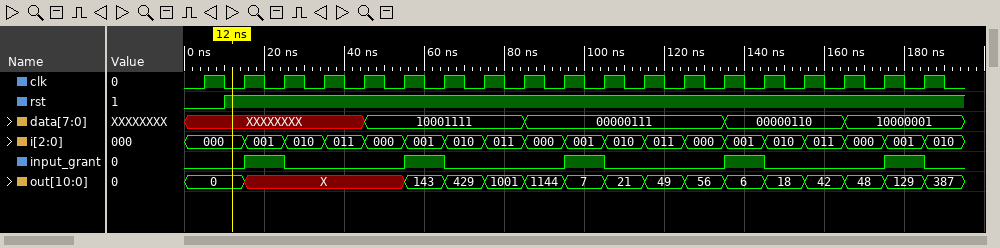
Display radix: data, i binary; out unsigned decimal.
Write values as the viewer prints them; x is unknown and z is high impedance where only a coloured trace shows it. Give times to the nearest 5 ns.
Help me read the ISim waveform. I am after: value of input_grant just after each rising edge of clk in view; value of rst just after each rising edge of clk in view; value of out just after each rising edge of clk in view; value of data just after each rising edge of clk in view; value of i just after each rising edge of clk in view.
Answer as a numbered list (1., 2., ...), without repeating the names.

1. 0 1 0 0 0 1 0 0 0 1 0 0 0 1 0 0 0 1 0
2. 0 1 1 1 1 1 1 1 1 1 1 1 1 1 1 1 1 1 1
3. 0, X, X, X, X, 143, 429, 1001, 1144, 7, 21, 49, 56, 6, 18, 42, 48, 129, 387
4. XXXXXXXX, XXXXXXXX, XXXXXXXX, XXXXXXXX, 10001111, 10001111, 10001111, 10001111, 00000111, 00000111, 00000111, 00000111, 00000111, 00000110, 00000110, 00000110, 10000001, 10000001, 10000001
5. 000, 001, 010, 011, 000, 001, 010, 011, 000, 001, 010, 011, 000, 001, 010, 011, 000, 001, 010
